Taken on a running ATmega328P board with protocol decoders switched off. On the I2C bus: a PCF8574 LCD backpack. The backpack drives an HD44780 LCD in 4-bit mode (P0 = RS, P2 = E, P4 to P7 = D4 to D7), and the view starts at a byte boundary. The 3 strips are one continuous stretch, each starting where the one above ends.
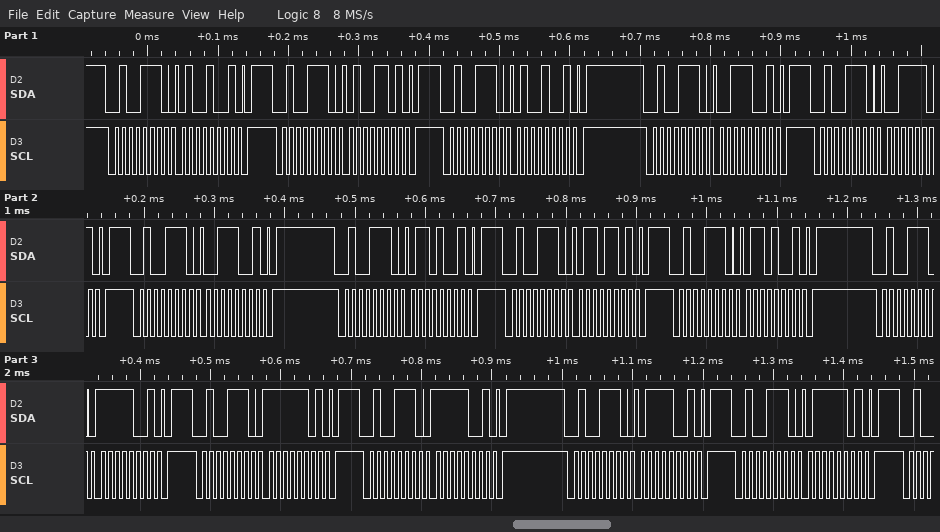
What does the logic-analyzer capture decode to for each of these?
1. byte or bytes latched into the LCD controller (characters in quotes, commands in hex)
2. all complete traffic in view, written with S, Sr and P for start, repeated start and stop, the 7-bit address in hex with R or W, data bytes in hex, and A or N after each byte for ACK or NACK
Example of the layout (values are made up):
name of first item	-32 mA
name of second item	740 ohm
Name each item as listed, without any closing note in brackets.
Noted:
byte or bytes latched into the LCD controller	'C' 'o'
all complete traffic in view, written with S, Sr and P for start, repeated start and stop, the 7-bit address in hex with R or W, data bytes in hex, and A or N after each byte for ACK or NACK	S 27W A 49 A P S 27W A 4D A P S 27W A 49 A P S 27W A 39 A P S 27W A 3D A P S 27W A 39 A P S 27W A 69 A P S 27W A 6D A P S 27W A 69 A P S 27W A F9 A P S 27W A FD A P S 27W A F9 A P S 27W A 79 A P S 27W A 7D A P
